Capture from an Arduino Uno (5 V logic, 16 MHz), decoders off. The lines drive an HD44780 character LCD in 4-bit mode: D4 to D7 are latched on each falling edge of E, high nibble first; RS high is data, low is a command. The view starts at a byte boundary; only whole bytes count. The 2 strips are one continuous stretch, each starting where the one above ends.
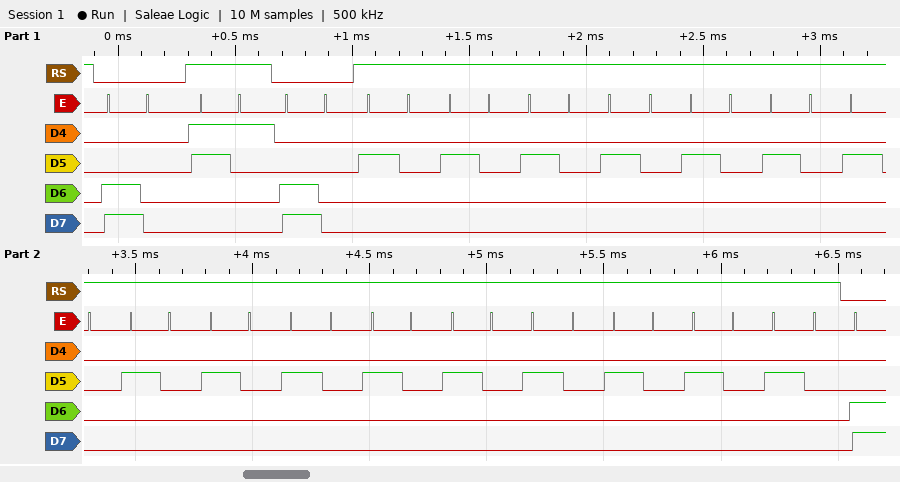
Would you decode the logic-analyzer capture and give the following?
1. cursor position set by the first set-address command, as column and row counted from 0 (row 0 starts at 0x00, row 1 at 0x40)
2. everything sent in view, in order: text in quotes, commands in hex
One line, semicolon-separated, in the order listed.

column 0, row 1; 0xC0 "1" 0xC0 "                "
